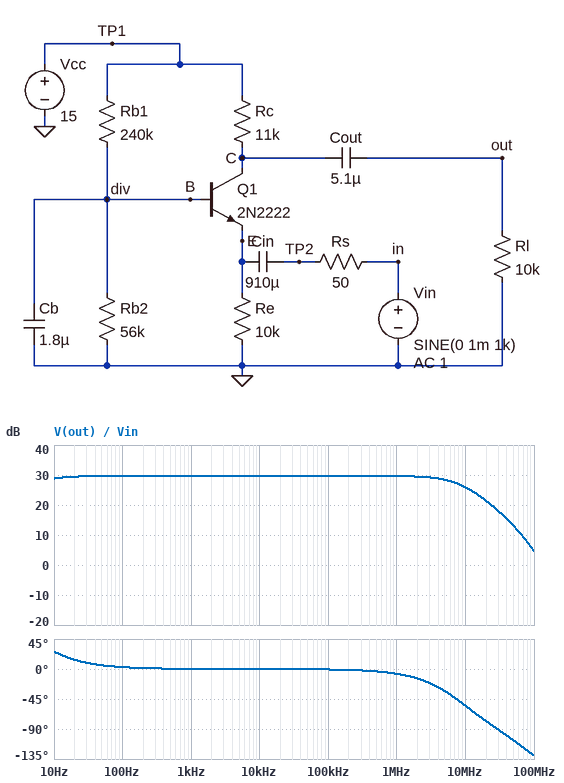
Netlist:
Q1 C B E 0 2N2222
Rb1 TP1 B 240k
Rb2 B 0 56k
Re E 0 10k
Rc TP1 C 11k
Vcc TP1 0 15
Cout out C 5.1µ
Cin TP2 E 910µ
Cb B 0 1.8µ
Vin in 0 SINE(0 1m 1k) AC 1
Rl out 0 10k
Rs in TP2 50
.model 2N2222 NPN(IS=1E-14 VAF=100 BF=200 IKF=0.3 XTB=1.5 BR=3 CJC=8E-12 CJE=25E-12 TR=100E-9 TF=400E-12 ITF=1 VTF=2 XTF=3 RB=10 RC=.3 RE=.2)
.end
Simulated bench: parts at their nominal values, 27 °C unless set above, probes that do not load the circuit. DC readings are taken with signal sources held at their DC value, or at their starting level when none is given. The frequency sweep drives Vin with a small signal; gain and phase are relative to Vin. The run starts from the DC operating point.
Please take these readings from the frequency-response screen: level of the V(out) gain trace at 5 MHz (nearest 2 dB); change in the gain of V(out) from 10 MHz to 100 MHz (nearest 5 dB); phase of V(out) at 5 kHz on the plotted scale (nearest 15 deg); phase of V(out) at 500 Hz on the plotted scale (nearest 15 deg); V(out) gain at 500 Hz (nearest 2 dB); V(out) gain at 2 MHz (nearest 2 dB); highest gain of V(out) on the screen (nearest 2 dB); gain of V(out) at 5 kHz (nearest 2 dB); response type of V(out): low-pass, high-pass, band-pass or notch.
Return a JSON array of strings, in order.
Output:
["28 dB", "-20 dB", "0 deg", "0 deg", "30 dB", "30 dB", "30 dB", "30 dB", "low-pass"]
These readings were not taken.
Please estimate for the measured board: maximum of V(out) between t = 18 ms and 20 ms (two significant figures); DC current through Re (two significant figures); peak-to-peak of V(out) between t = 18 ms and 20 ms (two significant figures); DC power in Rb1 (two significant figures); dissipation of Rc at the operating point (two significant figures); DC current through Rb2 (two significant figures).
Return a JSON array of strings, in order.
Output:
["30 mV", "220 µA", "61 mV", "620 µW", "520 µW", "50 µA"]
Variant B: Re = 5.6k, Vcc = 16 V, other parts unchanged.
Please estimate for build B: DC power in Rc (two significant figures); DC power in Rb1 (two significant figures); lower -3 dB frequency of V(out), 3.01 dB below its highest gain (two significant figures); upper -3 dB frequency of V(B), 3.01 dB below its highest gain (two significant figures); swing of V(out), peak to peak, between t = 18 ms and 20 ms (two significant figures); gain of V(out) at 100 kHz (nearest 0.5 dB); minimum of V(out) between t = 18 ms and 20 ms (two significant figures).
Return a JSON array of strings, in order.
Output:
["1.9 mW", "710 µW", "6.5 Hz", "7.5 Hz", "91 mV", "33.0 dB", "-46 mV"]
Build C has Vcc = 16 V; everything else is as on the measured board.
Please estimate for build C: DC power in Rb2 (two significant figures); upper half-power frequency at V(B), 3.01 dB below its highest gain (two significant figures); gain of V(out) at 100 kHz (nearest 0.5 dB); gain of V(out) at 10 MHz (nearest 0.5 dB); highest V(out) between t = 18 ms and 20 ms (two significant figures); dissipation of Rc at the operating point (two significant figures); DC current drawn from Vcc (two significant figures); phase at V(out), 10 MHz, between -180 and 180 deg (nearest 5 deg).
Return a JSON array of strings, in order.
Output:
["160 µW", "5.9 Hz", "30.0 dB", "26.5 dB", "32 mV", "610 µW", "290 µA", "-55 deg"]
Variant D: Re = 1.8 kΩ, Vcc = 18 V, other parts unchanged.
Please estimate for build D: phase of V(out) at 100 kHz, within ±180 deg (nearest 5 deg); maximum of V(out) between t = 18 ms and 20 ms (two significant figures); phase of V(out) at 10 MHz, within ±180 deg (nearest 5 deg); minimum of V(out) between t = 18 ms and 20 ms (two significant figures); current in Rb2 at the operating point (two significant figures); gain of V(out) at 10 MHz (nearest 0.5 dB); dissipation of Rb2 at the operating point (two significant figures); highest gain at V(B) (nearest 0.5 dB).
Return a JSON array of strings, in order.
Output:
["0 deg", "73 mV", "-75 deg", "-73 mV", "55 µA", "27.5 dB", "170 µW", "-4.5 dB"]
